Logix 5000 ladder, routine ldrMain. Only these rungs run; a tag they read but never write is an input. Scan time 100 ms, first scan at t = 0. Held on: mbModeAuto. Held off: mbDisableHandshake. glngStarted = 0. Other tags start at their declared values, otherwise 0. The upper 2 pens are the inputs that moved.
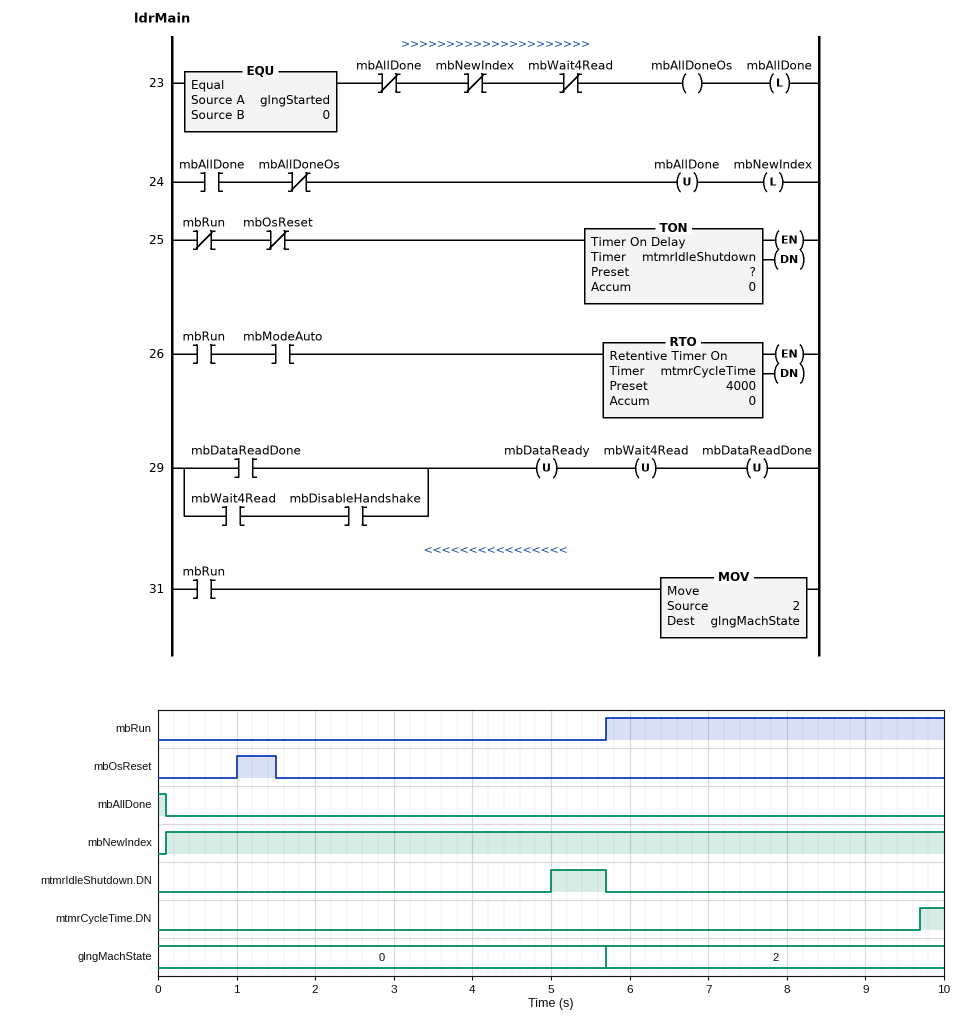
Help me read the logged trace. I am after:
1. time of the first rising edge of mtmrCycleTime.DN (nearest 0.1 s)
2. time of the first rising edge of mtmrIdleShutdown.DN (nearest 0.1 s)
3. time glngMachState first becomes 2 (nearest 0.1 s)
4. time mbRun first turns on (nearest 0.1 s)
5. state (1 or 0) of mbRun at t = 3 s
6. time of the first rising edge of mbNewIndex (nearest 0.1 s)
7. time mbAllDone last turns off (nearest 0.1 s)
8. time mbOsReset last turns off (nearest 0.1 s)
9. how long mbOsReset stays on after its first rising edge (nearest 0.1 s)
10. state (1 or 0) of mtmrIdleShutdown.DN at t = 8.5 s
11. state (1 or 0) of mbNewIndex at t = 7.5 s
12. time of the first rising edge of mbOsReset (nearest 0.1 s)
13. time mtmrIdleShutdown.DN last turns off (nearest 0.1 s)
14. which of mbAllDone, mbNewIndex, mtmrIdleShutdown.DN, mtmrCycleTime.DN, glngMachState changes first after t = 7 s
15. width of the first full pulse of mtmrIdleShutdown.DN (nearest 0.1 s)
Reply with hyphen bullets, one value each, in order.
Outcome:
- 9.7 s
- 5.0 s
- 5.7 s
- 5.7 s
- 0
- 0.1 s
- 0.1 s
- 1.5 s
- 0.5 s
- 0
- 1
- 1.0 s
- 5.7 s
- mtmrCycleTime.DN
- 0.7 s
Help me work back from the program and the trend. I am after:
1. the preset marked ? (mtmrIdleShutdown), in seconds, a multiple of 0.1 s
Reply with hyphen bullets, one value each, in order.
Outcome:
- 3.5 s
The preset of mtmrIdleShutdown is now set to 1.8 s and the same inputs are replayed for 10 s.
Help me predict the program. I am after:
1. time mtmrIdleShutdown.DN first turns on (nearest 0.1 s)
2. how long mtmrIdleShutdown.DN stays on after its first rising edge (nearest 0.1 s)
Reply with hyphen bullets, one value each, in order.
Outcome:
- 3.3 s
- 2.4 s
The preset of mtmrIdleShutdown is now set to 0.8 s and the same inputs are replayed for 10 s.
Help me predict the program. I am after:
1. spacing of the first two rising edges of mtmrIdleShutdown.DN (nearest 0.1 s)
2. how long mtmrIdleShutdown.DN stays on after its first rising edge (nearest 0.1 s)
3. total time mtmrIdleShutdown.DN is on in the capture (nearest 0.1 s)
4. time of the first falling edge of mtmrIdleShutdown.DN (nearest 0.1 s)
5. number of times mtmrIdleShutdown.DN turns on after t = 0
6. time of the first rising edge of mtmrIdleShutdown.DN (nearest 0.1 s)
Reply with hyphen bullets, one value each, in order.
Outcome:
- 1.5 s
- 0.2 s
- 3.6 s
- 1.0 s
- 2
- 0.8 s
